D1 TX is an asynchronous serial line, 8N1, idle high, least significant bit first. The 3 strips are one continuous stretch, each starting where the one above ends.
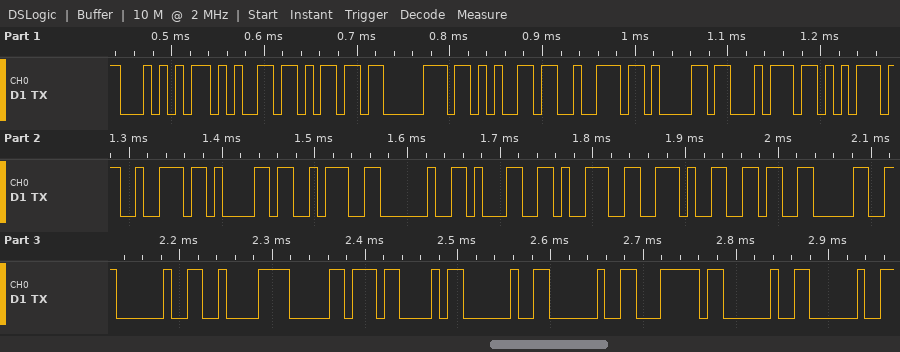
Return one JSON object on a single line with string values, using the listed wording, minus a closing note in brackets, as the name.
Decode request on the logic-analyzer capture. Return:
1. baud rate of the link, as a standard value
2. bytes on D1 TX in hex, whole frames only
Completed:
{"baud rate of the link, as a standard value": "115200 baud", "bytes on D1 TX in hex, whole frames only": "54 65 6D 70 65 72 61 74 75 72 61 3A 20 31 39 2E 36 30 20 C2 B0 43 20 20 7C 20 20"}
